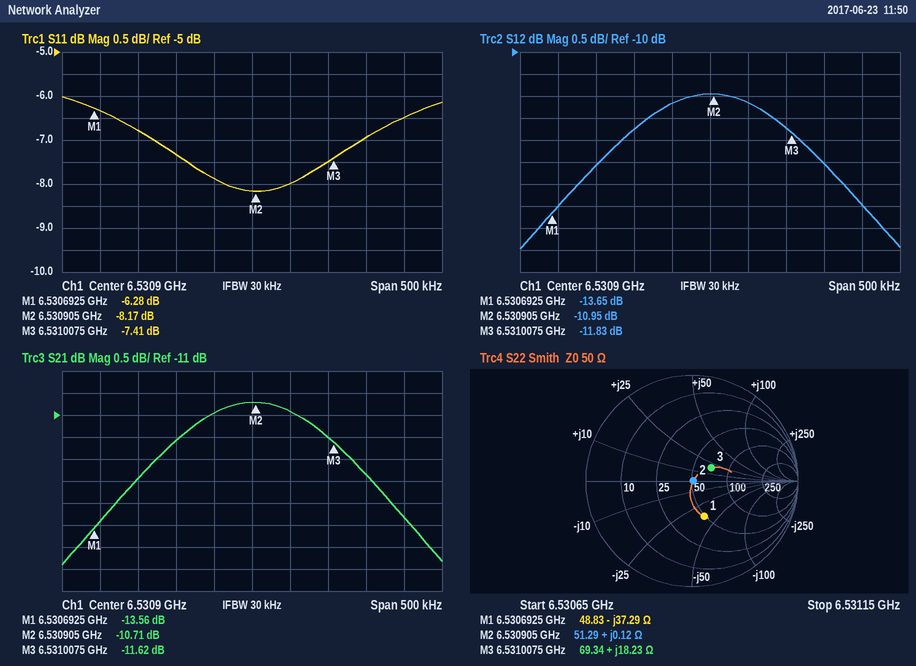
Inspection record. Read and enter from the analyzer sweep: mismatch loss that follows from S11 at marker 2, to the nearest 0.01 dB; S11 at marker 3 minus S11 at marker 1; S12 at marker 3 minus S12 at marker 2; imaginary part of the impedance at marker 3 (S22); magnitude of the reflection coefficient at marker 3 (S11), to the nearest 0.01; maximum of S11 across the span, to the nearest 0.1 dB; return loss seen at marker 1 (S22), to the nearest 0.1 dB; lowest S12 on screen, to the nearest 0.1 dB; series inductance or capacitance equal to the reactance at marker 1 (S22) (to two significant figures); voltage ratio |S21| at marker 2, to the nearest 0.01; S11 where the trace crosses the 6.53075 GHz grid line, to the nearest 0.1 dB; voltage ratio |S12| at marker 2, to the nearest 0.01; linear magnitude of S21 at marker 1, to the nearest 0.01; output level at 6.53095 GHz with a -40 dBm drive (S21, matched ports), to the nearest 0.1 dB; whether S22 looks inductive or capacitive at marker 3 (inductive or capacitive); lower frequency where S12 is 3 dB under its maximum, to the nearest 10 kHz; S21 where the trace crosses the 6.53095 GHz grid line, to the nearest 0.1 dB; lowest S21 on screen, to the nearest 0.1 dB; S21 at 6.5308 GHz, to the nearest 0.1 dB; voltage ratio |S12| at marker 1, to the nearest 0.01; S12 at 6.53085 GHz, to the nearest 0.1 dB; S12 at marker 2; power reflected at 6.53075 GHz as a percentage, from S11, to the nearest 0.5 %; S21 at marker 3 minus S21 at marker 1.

0.72 dB
-1.13 dB
-0.88 dB
+18.23 Ω
0.43
-6.0 dB
9.0 dB
-14.5 dB
650 fF
0.29
-6.8 dB
0.28
0.21
-50.9 dBm
inductive
6.53068 GHz
-10.9 dB
-14.4 dB
-11.6 dB
0.21
-11.2 dB
-10.95 dB
21.0 %
1.94 dB
